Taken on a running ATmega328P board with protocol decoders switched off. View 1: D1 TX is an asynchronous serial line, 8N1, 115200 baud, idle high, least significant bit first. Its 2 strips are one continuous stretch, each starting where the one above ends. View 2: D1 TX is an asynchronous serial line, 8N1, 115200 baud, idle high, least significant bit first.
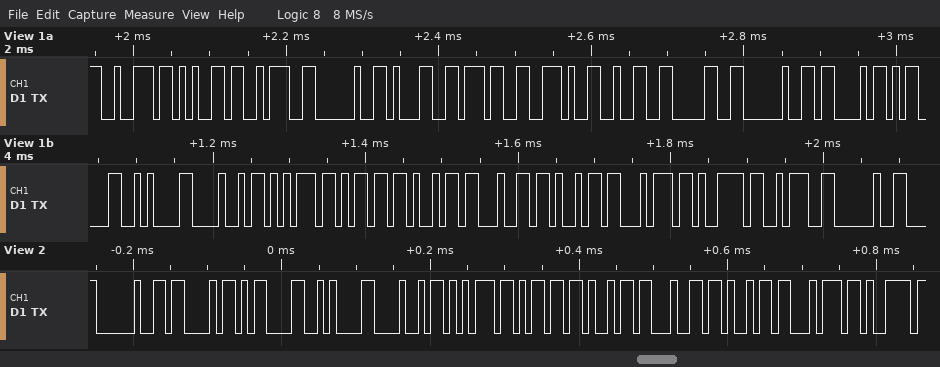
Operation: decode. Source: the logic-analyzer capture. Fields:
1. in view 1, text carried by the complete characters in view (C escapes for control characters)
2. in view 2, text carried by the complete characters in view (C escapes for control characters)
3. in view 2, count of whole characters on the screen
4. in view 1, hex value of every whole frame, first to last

"re: 17.20 C\r\nHumidity: "
" C\r\nHumidity"
12
72 65 3A 20 31 37 2E 32 30 20 43 0D 0A 48 75 6D 69 64 69 74 79 3A 20
